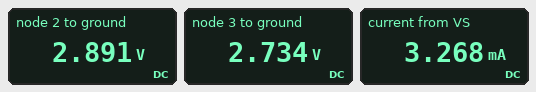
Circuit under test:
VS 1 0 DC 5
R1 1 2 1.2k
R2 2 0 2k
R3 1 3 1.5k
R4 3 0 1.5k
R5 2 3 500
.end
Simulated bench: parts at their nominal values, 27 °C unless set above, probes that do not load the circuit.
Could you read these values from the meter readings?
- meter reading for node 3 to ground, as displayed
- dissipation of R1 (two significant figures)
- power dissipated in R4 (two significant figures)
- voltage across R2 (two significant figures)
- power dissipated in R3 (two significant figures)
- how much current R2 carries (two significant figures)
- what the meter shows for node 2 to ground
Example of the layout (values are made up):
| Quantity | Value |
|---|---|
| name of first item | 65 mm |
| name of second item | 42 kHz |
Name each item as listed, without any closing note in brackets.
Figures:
| Quantity | Value |
|---|---|
| meter reading for node 3 to ground, as displayed | 2.734 V |
| dissipation of R1 | 3.7 mW |
| power dissipated in R4 | 5.0 mW |
| voltage across R2 | 2.9 V |
| power dissipated in R3 | 3.4 mW |
| how much current R2 carries | 1.4 mA |
| what the meter shows for node 2 to ground | 2.891 V |
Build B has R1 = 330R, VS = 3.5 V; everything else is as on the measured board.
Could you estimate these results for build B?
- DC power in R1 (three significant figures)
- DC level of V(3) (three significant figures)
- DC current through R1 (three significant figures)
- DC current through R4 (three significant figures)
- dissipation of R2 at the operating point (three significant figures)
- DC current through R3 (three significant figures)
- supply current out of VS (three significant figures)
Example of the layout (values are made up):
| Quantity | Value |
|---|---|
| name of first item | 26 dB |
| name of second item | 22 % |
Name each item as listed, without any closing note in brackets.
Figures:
| Quantity | Value |
|---|---|
| DC power in R1 | 1.60 mW |
| DC level of V(3) | 2.36 V |
| DC current through R1 | 2.20 mA |
| DC current through R4 | 1.58 mA |
| dissipation of R2 at the operating point | 3.84 mW |
| DC current through R3 | 758 µA |
| supply current out of VS | 2.96 mA |
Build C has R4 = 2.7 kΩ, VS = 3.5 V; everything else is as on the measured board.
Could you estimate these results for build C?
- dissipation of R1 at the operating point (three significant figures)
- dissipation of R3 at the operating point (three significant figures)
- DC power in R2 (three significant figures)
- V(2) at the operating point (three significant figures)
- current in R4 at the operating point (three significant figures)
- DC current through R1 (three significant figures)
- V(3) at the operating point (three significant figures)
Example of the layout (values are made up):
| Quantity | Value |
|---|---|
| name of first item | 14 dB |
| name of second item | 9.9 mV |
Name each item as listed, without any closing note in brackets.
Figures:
| Quantity | Value |
|---|---|
| dissipation of R1 at the operating point | 1.39 mW |
| dissipation of R3 at the operating point | 1.09 mW |
| DC power in R2 | 2.44 mW |
| V(2) at the operating point | 2.21 V |
| current in R4 at the operating point | 823 µA |
| DC current through R1 | 1.08 mA |
| V(3) at the operating point | 2.22 V |
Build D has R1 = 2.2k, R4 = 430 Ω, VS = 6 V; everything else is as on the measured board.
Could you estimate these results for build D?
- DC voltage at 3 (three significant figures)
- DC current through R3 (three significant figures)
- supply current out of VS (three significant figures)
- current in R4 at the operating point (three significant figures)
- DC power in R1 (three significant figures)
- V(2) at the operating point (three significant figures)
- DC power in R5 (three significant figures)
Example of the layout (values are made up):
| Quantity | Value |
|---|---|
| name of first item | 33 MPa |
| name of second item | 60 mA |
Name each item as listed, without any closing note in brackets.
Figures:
| Quantity | Value |
|---|---|
| DC voltage at 3 | 1.61 V |
| DC current through R3 | 2.93 mA |
| supply current out of VS | 4.74 mA |
| current in R4 at the operating point | 3.74 mA |
| DC power in R1 | 7.23 mW |
| V(2) at the operating point | 2.01 V |
| DC power in R5 | 326 µW |
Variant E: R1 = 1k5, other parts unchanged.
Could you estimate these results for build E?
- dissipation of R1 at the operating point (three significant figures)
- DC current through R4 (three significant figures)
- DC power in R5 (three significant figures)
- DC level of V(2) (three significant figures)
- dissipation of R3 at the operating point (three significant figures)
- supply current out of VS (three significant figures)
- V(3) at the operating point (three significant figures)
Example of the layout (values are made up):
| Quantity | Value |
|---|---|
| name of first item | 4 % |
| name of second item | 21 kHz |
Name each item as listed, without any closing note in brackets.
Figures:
| Quantity | Value |
|---|---|
| dissipation of R1 at the operating point | 3.49 mW |
| DC current through R4 | 1.75 mA |
| DC power in R5 | 14.4 µW |
| DC level of V(2) | 2.71 V |
| dissipation of R3 at the operating point | 3.75 mW |
| supply current out of VS | 3.11 mA |
| V(3) at the operating point | 2.63 V |
